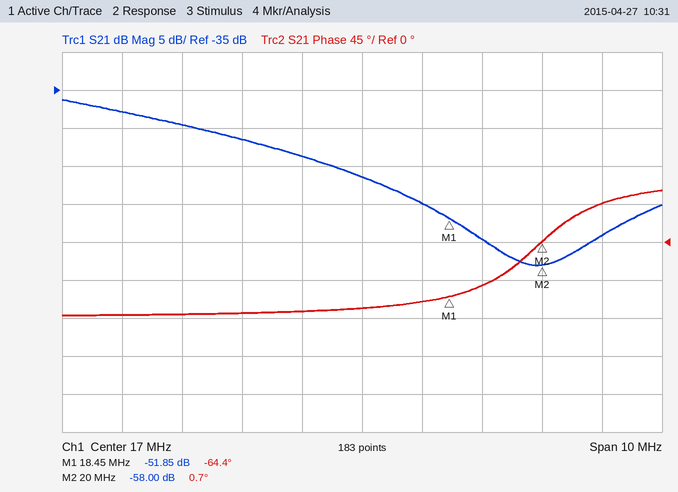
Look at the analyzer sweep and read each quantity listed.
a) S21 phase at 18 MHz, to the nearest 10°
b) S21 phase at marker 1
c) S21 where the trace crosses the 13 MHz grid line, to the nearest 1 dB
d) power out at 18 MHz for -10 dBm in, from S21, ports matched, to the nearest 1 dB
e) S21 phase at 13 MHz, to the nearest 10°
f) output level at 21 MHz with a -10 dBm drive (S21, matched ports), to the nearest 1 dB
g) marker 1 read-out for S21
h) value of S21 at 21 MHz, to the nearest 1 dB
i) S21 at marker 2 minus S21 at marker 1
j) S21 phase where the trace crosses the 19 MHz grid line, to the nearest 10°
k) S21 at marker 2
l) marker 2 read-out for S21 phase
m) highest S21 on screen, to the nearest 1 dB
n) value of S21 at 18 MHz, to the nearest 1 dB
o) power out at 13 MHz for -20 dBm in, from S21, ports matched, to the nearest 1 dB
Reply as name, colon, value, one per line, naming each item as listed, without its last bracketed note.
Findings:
S21 phase at 18 MHz, to the nearest 10°: -70°
S21 phase at marker 1: -64.4°
S21 where the trace crosses the 13 MHz grid line, to the nearest 1 dB: -38 dB
power out at 18 MHz for -10 dBm in, from S21, ports matched, to the nearest 1 dB: -60 dBm
S21 phase at 13 MHz, to the nearest 10°: -90°
output level at 21 MHz with a -10 dBm drive (S21, matched ports), to the nearest 1 dB: -64 dBm
marker 1 read-out for S21: -51.85 dB
value of S21 at 21 MHz, to the nearest 1 dB: -54 dB
S21 at marker 2 minus S21 at marker 1: -6.15 dB
S21 phase where the trace crosses the 19 MHz grid line, to the nearest 10°: -50°
S21 at marker 2: -58.00 dB
marker 2 read-out for S21 phase: 0.7°
highest S21 on screen, to the nearest 1 dB: -36 dB
value of S21 at 18 MHz, to the nearest 1 dB: -50 dB
power out at 13 MHz for -20 dBm in, from S21, ports matched, to the nearest 1 dB: -58 dBm
